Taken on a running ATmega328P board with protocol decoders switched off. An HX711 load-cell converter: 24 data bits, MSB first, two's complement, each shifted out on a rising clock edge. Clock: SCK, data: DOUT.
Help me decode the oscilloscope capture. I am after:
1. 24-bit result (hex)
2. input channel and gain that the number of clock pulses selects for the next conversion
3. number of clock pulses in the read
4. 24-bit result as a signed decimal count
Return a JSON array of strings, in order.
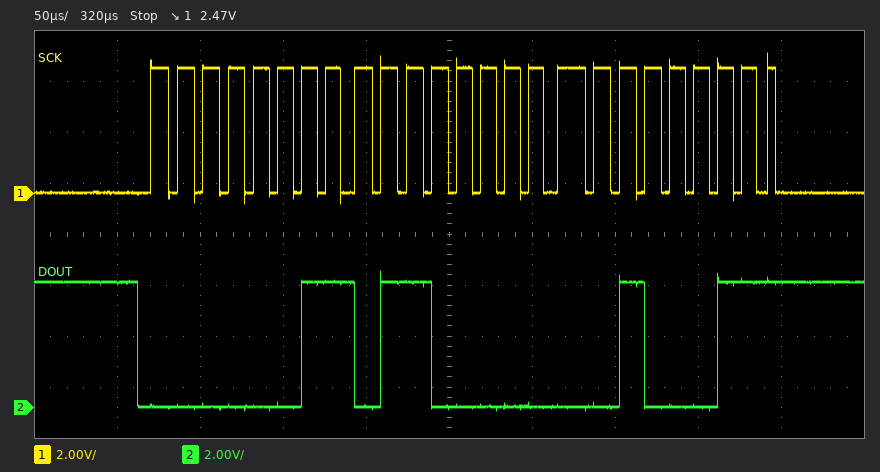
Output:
["0x036023", "channel A, gain 128", "25", "221219"]
